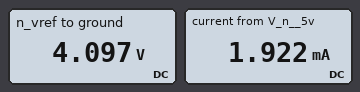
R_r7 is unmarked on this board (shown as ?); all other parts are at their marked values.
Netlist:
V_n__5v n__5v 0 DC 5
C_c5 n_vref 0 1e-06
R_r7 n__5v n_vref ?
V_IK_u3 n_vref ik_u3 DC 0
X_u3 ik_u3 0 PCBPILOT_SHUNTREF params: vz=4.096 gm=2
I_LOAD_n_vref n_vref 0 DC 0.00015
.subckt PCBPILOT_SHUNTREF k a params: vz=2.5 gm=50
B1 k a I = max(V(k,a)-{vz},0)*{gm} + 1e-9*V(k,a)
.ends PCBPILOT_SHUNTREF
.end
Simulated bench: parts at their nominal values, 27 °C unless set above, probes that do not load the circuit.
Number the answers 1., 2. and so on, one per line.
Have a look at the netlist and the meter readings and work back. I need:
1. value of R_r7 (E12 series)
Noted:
1. 470 Ω
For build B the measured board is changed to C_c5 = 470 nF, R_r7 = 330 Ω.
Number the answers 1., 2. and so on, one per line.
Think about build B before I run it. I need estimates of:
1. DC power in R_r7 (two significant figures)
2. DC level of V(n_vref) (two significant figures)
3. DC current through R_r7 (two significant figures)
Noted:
1. 2.5 mW
2. 4.1 V
3. 2.7 mA
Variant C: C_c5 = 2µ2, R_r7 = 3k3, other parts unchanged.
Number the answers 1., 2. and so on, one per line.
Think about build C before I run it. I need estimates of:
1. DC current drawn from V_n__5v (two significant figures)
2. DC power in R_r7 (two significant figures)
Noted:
1. 270 µA
2. 250 µW
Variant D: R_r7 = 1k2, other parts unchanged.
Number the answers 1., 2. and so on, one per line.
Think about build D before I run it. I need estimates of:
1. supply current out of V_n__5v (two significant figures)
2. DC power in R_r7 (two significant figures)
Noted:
1. 750 µA
2. 680 µW
